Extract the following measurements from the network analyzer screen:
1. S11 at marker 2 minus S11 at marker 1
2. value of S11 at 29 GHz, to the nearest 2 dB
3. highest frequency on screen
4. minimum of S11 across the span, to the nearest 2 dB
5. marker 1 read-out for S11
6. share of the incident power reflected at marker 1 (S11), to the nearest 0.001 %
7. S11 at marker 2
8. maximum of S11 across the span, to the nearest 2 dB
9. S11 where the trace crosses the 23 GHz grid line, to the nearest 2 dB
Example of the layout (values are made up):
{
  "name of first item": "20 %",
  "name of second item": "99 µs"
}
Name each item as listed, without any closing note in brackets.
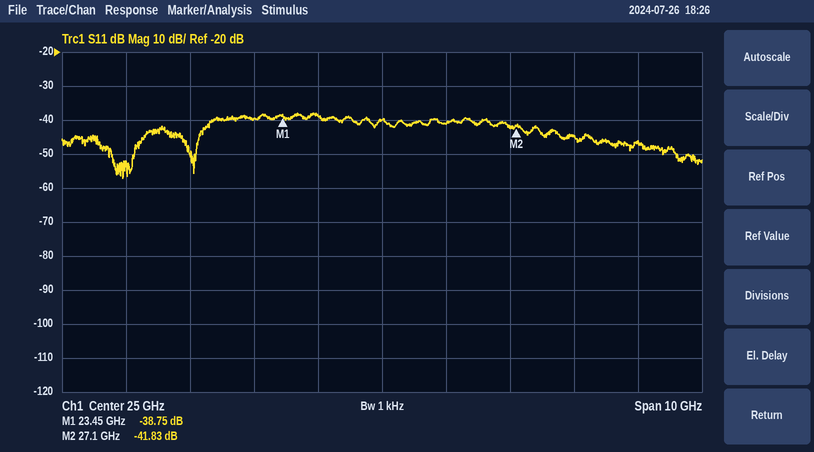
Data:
{
  "S11 at marker 2 minus S11 at marker 1": "-3.08 dB",
  "value of S11 at 29 GHz, to the nearest 2 dB": "-46 dB",
  "highest frequency on screen": "30 GHz",
  "minimum of S11 across the span, to the nearest 2 dB": "-58 dB",
  "marker 1 read-out for S11": "-38.75 dB",
  "share of the incident power reflected at marker 1 (S11), to the nearest 0.001 %": "0.013 %",
  "S11 at marker 2": "-41.83 dB",
  "maximum of S11 across the span, to the nearest 2 dB": "-38 dB",
  "S11 where the trace crosses the 23 GHz grid line, to the nearest 2 dB": "-40 dB"
}
